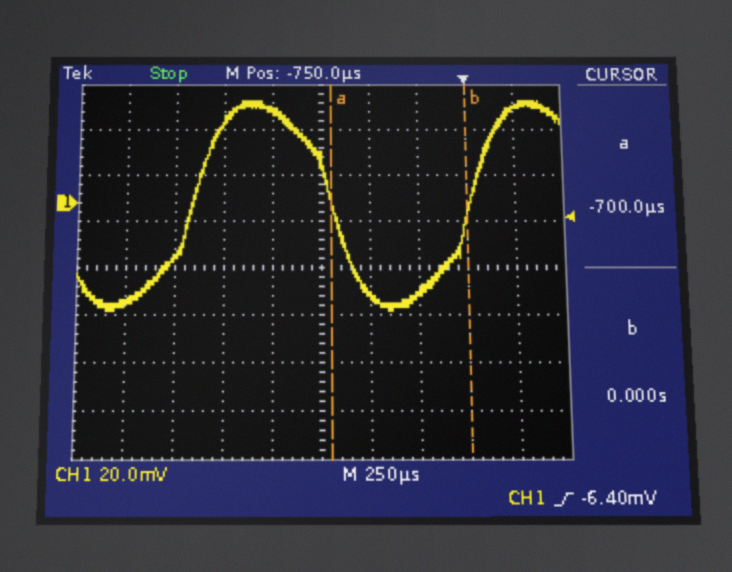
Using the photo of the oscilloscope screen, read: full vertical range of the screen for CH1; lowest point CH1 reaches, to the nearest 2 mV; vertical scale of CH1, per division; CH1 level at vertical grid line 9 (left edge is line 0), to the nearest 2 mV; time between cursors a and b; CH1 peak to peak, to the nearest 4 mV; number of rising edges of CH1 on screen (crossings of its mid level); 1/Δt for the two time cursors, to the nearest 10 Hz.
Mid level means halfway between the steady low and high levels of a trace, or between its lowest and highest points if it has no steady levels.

160 mV
-46 mV
20 mV
42 mV
700 µs
92 mV
2
1.43 kHz
